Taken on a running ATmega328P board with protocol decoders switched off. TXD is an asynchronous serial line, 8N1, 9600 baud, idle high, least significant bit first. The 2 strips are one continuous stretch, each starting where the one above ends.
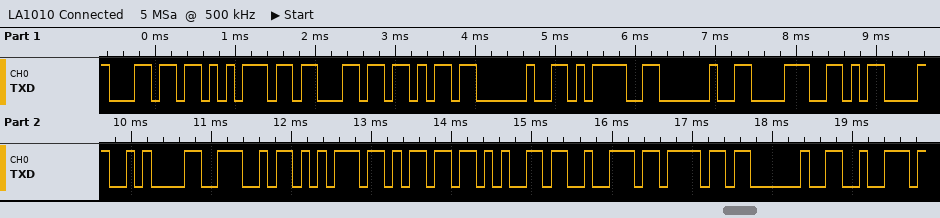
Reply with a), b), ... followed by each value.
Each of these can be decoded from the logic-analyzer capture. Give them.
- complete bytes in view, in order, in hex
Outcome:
a) 6C 75 63 6B 20 3D 20 38 0D 0A 4E 75 6D 65 72 6F 20 72
